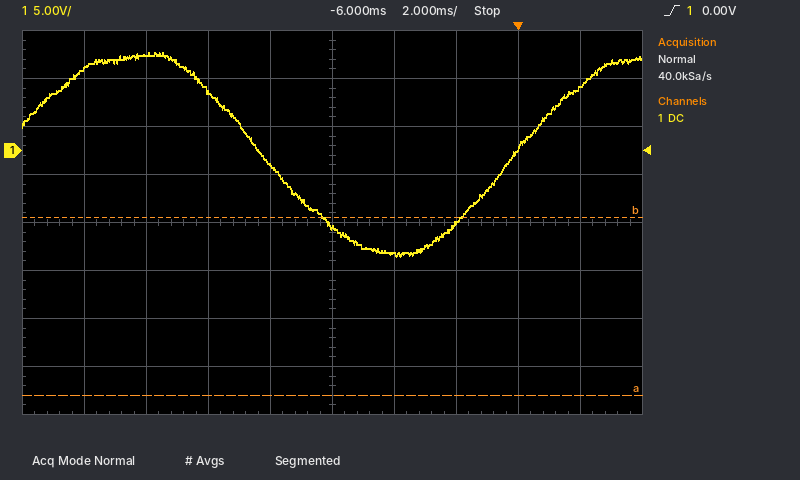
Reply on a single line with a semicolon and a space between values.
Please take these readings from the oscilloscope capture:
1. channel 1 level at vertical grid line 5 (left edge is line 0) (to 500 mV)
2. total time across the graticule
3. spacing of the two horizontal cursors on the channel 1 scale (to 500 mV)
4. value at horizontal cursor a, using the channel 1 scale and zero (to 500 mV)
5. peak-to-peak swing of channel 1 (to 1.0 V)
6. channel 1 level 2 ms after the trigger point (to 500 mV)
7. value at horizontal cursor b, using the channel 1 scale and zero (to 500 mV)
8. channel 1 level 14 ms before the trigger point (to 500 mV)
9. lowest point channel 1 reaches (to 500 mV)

-8.0 V; 20 ms; 18.5 V; -25.5 V; 21.0 V; 6.5 V; -7.0 V; 8.5 V; -11.0 V
